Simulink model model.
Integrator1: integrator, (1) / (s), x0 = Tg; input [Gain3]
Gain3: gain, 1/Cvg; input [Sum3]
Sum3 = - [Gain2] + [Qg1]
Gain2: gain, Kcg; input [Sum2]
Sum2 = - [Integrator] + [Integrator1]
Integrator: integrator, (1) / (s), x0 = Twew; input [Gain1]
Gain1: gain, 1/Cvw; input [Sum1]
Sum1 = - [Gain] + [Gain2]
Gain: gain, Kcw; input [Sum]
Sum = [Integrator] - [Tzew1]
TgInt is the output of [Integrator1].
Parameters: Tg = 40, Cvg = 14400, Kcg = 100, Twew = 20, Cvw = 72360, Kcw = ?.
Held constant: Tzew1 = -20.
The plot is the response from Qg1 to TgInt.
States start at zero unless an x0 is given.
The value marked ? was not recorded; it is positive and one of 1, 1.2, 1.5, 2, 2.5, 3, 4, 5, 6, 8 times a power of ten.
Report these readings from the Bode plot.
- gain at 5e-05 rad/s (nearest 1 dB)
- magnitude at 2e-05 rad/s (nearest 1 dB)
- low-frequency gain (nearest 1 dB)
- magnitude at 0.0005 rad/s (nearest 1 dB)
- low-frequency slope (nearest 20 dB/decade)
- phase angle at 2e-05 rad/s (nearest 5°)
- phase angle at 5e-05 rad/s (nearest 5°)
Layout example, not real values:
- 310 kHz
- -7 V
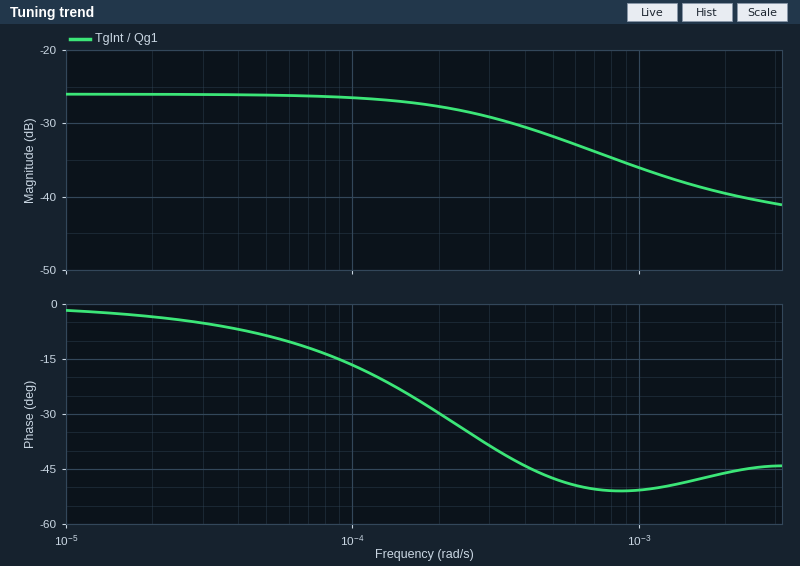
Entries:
- -26 dB
- -26 dB
- -26 dB
- -32 dB
- 0 dB/decade
- -5°
- -10°
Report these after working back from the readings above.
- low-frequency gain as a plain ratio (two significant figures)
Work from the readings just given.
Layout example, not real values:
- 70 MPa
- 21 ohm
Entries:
- 0.050
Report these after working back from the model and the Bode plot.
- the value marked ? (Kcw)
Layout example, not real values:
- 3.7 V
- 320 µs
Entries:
- 25
